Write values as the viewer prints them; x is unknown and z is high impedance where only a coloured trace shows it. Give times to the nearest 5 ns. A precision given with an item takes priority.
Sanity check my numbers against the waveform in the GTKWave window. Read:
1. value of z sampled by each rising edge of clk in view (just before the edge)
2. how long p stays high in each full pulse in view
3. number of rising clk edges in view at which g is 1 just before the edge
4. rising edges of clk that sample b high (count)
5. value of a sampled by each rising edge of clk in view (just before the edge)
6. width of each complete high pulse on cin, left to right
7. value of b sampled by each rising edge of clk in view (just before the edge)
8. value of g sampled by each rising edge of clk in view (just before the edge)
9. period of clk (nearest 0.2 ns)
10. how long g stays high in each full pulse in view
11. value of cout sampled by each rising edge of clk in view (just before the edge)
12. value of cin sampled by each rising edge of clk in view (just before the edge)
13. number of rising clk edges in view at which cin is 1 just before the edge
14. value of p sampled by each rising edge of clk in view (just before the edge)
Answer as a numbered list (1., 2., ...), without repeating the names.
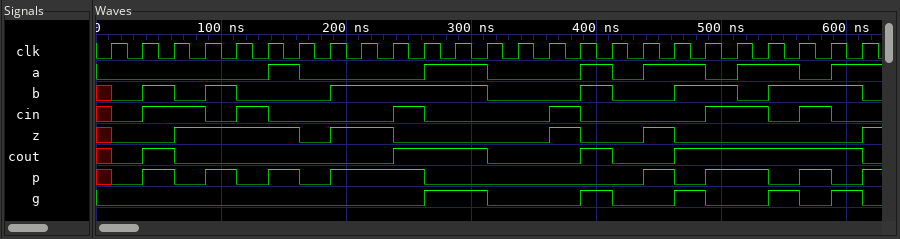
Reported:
1. x 0 0 1 1 1 1 0 1 1 0 0 0 0 0 1 0 0 1 0 0 0 0 0 0
2. 25 ns, 25 ns, 25 ns, 75 ns, 25 ns, 50 ns, 25 ns
3. 6
4. 13
5. 0 0 0 0 0 0 1 0 0 0 0 1 1 0 0 0 1 0 1 1 0 1 1 0 1
6. 50 ns, 25 ns, 25 ns, 25 ns, 50 ns, 25 ns
7. x 0 1 0 1 0 0 0 1 1 1 1 1 0 0 0 1 0 0 1 1 0 1 1 1
8. 0 0 0 0 0 0 0 0 0 0 0 1 1 0 0 0 1 0 0 1 0 0 1 0 1
9. 25 ns
10. 50 ns, 25 ns, 25 ns, 25 ns, 25 ns
11. x 0 1 0 0 0 0 0 0 0 1 1 1 0 0 0 1 0 0 1 1 1 1 1 1
12. x 0 1 1 0 1 0 0 0 0 1 0 0 0 0 1 0 0 0 0 1 1 0 1 0
13. 8
14. x 0 1 0 1 0 1 0 1 1 1 0 0 0 0 0 0 0 1 0 1 1 0 1 0
